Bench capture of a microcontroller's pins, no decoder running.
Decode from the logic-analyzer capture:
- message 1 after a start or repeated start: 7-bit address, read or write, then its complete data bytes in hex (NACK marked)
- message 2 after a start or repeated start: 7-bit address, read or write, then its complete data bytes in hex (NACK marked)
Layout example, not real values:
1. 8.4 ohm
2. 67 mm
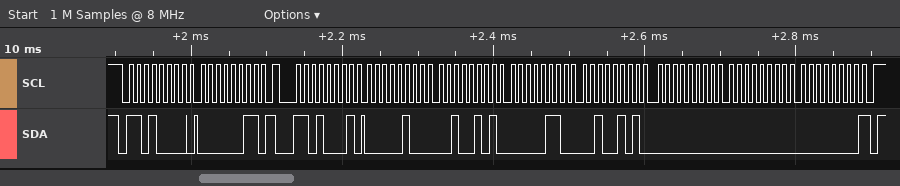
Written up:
1. 0x68 write: 03
2. 0x68 read: 04 25 06 25 00 00 00 NACK
